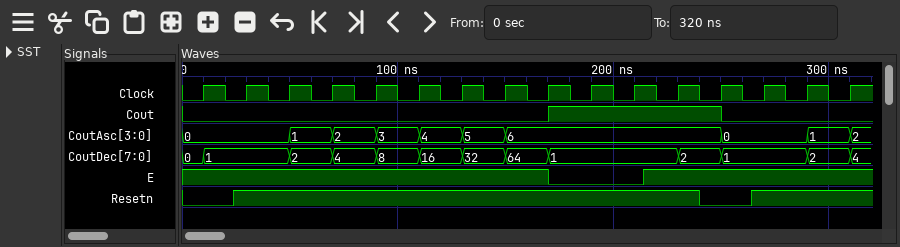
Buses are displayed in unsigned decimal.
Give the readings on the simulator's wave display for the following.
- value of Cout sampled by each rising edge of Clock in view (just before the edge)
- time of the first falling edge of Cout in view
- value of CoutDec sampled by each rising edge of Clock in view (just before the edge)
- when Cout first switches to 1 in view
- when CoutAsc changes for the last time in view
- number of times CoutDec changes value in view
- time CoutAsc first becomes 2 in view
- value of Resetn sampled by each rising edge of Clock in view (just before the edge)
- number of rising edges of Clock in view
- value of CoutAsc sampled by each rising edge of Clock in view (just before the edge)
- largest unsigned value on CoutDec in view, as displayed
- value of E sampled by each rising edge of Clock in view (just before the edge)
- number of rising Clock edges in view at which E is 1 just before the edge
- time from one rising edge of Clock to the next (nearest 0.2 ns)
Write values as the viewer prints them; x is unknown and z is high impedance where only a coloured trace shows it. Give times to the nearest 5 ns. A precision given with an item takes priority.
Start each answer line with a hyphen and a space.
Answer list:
- 0 0 0 0 0 0 0 0 0 1 1 1 1 0 0 0
- 250 ns
- 0, 1, 1, 2, 4, 8, 16, 32, 64, 1, 1, 1, 2, 1, 1, 2
- 170 ns
- 310 ns
- 12
- 70 ns
- 0 1 1 1 1 1 1 1 1 1 1 1 0 1 1 1
- 16
- 0, 0, 0, 1, 2, 3, 4, 5, 6, 6, 6, 6, 6, 0, 0, 1
- 64
- 1 1 1 1 1 1 1 1 1 0 0 1 1 1 1 1
- 14
- 20 ns
